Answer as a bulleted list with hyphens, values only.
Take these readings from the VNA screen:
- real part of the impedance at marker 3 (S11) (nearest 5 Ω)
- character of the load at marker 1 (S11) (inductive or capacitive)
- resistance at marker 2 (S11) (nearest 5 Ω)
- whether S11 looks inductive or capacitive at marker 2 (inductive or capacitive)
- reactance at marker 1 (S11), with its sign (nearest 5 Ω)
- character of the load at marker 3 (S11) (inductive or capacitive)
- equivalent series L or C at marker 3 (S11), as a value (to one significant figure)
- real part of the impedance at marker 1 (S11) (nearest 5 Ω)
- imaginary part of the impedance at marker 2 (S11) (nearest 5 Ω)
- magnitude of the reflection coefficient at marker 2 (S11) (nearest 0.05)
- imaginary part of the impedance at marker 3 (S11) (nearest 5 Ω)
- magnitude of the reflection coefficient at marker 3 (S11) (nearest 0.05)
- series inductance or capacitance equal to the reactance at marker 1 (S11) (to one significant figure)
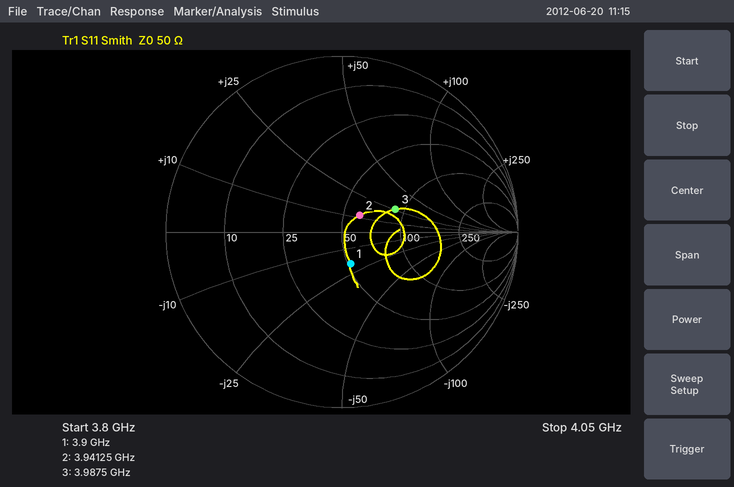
- 90 Ω
- capacitive
- 60 Ω
- inductive
- -20 Ω
- inductive
- 1 nH
- 50 Ω
- +10 Ω
- 0.15
- +25 Ω
- 0.35
- 2 pF
